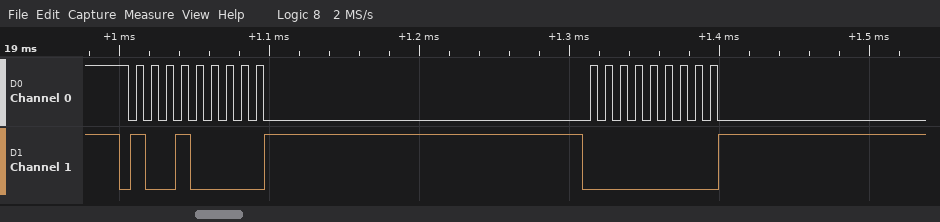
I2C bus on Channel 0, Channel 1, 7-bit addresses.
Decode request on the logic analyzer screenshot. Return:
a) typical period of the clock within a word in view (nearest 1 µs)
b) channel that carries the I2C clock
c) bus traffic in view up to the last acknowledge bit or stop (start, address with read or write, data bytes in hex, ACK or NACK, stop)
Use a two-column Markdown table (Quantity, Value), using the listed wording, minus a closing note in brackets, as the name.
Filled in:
| Quantity | Value |
|---|---|
| typical period of the clock within a word in view | 10 µs |
| channel that carries the I2C clock | Channel 0 |
| bus traffic in view up to the last acknowledge bit or stop | start, address 48 write ACK, 00 ACK |
